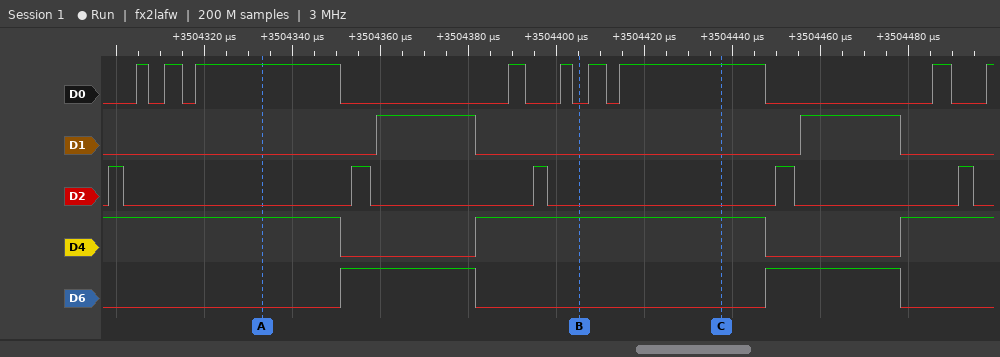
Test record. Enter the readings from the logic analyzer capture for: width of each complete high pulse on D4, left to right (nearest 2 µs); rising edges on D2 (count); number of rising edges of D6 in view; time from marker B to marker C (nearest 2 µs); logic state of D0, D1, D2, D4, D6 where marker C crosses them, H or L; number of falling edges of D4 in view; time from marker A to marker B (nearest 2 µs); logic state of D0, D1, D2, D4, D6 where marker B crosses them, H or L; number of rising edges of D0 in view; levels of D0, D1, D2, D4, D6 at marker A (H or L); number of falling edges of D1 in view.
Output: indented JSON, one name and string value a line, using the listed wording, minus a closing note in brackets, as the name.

{
  "width of each complete high pulse on D4, left to right": "66 µs",
  "rising edges on D2": "5",
  "number of rising edges of D6 in view": "2",
  "time from marker B to marker C": "32 µs",
  "logic state of D0, D1, D2, D4, D6 where marker C crosses them, H or L": "D0=H, D1=L, D2=L, D4=H, D6=L",
  "number of falling edges of D4 in view": "2",
  "time from marker A to marker B": "72 µs",
  "logic state of D0, D1, D2, D4, D6 where marker B crosses them, H or L": "D0=L, D1=L, D2=L, D4=H, D6=L",
  "number of rising edges of D0 in view": "9",
  "levels of D0, D1, D2, D4, D6 at marker A": "D0=H, D1=L, D2=L, D4=H, D6=L",
  "number of falling edges of D1 in view": "2"
}
